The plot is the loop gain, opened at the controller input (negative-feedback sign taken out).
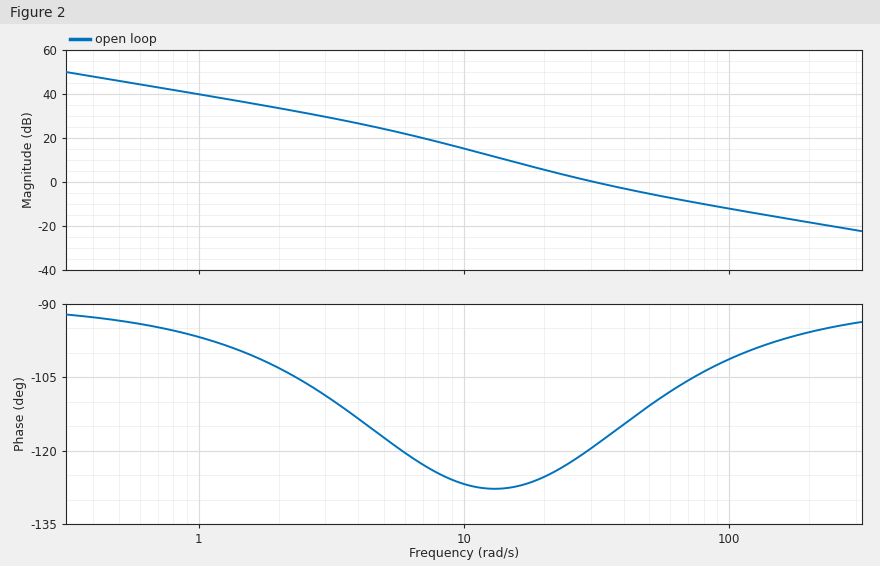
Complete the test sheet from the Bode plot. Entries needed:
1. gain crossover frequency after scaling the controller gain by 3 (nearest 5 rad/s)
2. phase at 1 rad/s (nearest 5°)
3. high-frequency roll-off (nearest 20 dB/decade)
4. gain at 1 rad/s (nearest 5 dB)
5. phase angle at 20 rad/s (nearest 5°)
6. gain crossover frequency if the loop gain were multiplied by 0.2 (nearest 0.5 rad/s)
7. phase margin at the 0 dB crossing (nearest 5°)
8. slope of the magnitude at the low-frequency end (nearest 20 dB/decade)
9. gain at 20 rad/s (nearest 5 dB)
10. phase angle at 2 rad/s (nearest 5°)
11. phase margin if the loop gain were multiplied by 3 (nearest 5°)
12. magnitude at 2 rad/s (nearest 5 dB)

75 rad/s
-95°
-20 dB/decade
40 dB
-125°
11.0 rad/s
60°
-20 dB/decade
5 dB
-105°
75°
35 dB
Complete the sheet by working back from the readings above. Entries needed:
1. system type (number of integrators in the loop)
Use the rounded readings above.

1
